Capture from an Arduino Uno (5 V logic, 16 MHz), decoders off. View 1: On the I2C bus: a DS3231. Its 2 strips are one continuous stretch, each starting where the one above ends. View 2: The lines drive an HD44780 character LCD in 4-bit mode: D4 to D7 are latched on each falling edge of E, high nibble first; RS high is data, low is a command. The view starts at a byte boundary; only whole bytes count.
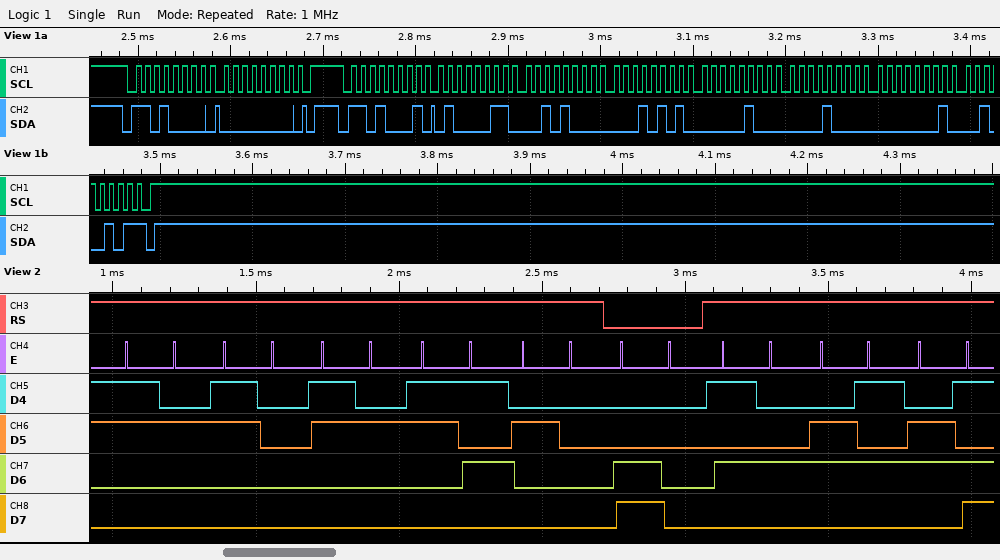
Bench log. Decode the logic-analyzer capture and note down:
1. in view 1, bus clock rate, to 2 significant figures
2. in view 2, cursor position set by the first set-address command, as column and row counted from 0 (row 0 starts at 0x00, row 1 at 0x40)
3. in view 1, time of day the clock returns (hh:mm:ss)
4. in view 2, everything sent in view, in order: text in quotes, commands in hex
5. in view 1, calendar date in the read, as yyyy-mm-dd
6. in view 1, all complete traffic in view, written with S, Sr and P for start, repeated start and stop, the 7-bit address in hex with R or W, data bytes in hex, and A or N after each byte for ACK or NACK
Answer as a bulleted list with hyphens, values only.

- 100 kHz
- column 0, row 1
- 15:28:43
- "2025 " 0xC0 "Tem"
- 2025-01-08
- S 68W A 00 A P S 68R A 43 A 28 A 15 A 04 A 08 A 01 A 25 N P
